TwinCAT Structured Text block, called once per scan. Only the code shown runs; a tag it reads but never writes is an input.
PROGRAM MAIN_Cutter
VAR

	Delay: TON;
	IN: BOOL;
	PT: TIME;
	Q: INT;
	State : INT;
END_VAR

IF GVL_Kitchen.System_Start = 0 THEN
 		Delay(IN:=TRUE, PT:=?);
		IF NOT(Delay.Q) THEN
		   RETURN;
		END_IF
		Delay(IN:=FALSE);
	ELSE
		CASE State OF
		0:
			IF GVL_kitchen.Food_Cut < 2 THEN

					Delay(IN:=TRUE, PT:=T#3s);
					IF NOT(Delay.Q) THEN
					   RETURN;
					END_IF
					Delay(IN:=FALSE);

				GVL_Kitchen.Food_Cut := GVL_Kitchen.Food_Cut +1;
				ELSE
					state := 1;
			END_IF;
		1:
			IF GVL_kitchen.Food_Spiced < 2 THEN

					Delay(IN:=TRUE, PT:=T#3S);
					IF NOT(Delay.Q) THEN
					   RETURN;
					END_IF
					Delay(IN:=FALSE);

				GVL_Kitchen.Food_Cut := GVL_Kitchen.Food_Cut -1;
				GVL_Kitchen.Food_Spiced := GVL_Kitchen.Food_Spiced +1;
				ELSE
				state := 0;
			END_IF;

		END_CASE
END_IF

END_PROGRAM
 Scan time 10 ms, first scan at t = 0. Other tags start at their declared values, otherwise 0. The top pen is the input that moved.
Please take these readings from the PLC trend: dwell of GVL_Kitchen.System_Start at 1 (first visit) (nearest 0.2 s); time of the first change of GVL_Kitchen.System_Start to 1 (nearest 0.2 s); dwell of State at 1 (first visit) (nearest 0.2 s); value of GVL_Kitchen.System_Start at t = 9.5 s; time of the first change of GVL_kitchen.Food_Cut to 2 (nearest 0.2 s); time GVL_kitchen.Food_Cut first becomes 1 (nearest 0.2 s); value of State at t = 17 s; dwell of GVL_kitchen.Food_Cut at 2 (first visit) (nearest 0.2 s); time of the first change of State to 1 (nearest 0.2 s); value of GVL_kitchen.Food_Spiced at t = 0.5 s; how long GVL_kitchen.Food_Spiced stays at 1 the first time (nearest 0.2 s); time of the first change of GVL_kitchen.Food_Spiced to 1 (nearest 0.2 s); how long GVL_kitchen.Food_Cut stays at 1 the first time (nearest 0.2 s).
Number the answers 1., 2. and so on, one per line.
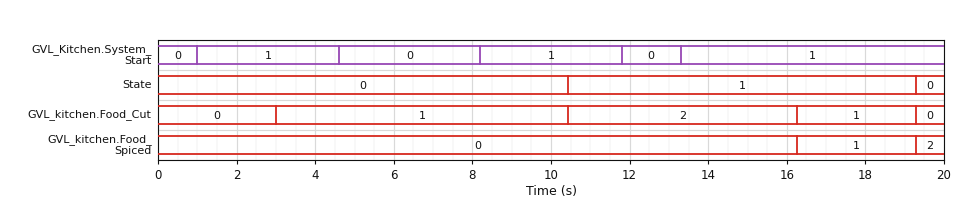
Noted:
1. 3.6 s
2. 1.0 s
3. 8.8 s
4. 1
5. 10.4 s
6. 3.0 s
7. 1
8. 5.8 s
9. 10.4 s
10. 0
11. 3.0 s
12. 16.2 s
13. 7.4 s
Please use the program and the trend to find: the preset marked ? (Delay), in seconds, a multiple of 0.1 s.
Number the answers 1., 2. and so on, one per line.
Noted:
1. 1.4 s
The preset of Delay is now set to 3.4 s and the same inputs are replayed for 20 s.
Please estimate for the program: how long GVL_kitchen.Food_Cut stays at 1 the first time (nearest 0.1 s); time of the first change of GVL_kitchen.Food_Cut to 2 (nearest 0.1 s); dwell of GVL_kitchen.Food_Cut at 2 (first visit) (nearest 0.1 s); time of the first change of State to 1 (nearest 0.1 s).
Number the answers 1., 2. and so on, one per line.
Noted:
1. 6.4 s
2. 9.4 s
3. 6.4 s
4. 9.4 s
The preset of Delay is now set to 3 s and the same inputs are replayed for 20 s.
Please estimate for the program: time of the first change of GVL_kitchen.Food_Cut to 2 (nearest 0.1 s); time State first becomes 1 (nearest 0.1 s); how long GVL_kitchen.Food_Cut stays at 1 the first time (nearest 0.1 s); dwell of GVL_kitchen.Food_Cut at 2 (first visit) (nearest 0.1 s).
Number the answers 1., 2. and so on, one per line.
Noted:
1. 9.0 s
2. 9.0 s
3. 6.0 s
4. 6.0 s
